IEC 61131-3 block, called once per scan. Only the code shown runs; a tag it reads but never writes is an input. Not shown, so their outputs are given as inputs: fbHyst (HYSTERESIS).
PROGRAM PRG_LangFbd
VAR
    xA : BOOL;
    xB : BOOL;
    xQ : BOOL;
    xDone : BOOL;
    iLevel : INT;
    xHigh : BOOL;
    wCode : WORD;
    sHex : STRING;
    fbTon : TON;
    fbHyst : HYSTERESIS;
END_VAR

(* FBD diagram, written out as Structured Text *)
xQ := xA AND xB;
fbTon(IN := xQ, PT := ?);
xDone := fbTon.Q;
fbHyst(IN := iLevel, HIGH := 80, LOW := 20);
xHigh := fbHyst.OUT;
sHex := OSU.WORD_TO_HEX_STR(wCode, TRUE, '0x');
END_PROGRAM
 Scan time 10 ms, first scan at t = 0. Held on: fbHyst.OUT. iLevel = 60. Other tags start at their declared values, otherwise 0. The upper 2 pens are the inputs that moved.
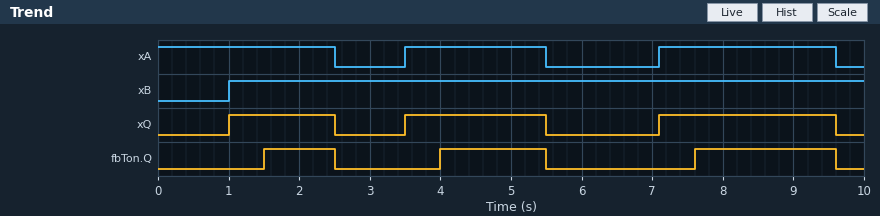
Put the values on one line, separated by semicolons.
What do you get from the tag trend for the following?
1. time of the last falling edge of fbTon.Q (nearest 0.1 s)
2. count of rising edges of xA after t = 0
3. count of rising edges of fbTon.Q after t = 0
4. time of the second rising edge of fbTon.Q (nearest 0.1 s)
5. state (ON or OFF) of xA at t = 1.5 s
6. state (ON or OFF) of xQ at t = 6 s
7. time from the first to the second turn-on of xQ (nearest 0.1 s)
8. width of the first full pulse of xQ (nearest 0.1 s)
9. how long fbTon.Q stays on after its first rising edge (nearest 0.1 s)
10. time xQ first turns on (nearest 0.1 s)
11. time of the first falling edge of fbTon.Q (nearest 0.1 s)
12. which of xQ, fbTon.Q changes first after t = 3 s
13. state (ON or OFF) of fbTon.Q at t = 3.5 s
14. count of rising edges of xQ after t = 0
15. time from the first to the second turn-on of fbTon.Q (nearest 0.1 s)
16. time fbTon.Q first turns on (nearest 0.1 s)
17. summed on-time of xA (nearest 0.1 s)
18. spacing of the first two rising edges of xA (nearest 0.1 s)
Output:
9.6 s; 2; 3; 4.0 s; ON; OFF; 2.5 s; 1.5 s; 1.0 s; 1.0 s; 2.5 s; xQ; OFF; 3; 2.5 s; 1.5 s; 7.0 s; 3.6 s
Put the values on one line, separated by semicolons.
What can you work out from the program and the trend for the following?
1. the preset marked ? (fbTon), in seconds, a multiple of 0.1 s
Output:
0.5 s
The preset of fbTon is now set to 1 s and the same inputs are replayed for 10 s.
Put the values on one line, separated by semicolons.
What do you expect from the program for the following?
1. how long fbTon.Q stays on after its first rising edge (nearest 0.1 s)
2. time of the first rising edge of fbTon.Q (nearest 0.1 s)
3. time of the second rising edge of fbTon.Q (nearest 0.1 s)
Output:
0.5 s; 2.0 s; 4.5 s
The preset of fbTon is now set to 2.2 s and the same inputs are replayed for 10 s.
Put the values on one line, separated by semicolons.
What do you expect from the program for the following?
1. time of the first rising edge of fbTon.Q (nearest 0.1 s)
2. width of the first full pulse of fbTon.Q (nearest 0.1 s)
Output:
9.3 s; 0.3 s
